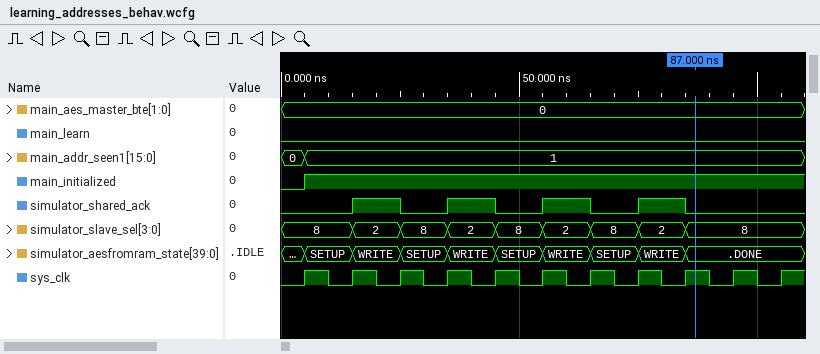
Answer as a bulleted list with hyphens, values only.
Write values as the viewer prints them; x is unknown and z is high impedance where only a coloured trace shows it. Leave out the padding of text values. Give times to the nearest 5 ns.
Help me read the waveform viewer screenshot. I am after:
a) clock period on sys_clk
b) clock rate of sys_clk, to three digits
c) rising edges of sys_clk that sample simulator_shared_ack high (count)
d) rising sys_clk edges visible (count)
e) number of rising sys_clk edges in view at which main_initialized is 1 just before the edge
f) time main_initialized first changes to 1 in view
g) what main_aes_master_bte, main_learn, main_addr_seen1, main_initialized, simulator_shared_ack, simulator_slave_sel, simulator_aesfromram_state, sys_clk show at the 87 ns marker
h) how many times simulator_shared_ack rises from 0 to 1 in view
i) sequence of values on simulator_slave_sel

- 10 ns
- 100 MHz
- 4
- 11
- 10
- 5 ns
- main_aes_master_bte=0, main_learn=0, main_addr_seen1=1, main_initialized=1, simulator_shared_ack=0, simulator_slave_sel=8, simulator_aesfromram_state=DONE, sys_clk=1
- 4
- 8, 2, 8, 2, 8, 2, 8, 2, 8
